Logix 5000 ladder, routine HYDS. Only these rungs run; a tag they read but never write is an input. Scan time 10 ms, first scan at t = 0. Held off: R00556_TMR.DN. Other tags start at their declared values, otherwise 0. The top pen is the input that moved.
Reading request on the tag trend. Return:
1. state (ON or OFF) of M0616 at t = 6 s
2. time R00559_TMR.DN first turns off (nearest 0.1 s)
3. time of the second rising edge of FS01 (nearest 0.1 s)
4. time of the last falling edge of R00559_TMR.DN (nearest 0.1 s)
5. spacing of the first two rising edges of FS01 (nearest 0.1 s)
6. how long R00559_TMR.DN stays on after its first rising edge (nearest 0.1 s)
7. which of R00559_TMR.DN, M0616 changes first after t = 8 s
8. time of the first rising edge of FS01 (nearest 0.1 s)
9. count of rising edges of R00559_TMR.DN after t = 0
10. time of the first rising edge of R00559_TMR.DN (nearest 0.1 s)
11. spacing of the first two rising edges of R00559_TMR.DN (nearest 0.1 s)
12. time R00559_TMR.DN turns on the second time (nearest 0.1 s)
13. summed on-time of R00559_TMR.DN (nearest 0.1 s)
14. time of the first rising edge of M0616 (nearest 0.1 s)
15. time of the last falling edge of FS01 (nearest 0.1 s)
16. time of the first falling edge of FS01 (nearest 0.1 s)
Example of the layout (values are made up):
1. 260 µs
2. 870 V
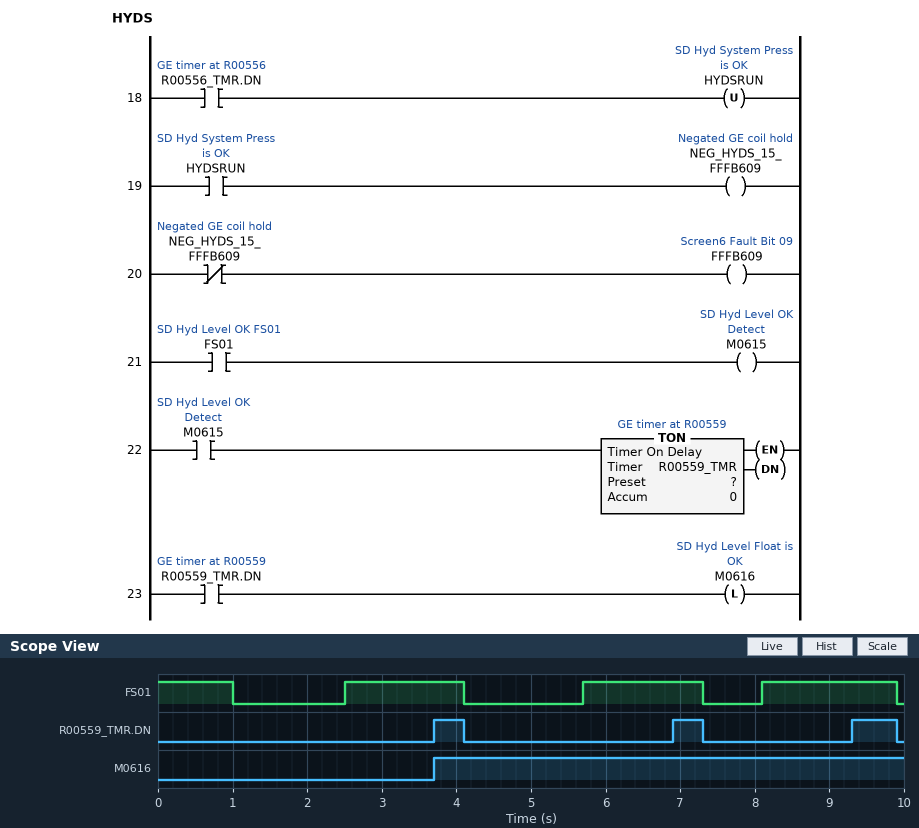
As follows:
1. ON
2. 4.1 s
3. 5.7 s
4. 9.9 s
5. 3.2 s
6. 0.4 s
7. R00559_TMR.DN
8. 2.5 s
9. 3
10. 3.7 s
11. 3.2 s
12. 6.9 s
13. 1.4 s
14. 3.7 s
15. 9.9 s
16. 1.0 s
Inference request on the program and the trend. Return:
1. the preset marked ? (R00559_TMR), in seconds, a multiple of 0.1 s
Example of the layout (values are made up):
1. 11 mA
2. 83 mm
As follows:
1. 1.2 s
